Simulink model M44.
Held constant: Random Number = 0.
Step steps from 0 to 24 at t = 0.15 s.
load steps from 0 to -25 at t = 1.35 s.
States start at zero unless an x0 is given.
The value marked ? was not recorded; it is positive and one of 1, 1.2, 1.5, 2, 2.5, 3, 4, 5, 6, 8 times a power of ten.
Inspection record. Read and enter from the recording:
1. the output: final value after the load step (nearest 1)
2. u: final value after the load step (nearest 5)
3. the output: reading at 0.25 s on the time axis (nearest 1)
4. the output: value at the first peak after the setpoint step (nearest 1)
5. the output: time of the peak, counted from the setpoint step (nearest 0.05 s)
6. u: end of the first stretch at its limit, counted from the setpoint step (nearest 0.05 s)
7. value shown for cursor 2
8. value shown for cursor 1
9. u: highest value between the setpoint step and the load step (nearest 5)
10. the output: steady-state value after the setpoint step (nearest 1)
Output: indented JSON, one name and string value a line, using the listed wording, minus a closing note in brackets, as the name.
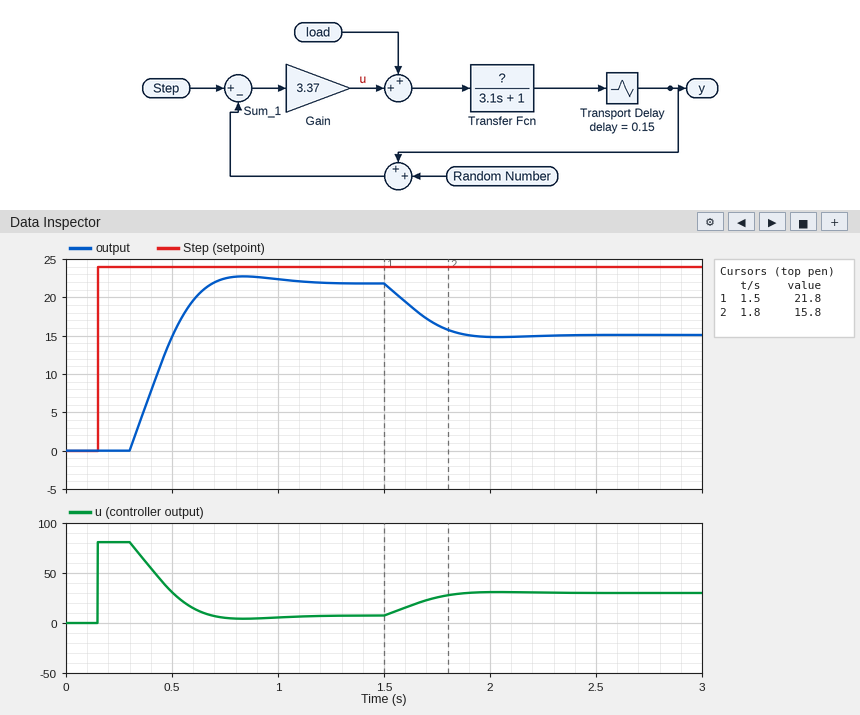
{
  "the output: final value after the load step": "15",
  "u: final value after the load step": "30",
  "the output: reading at 0.25 s on the time axis": "0",
  "the output: value at the first peak after the setpoint step": "23",
  "the output: time of the peak, counted from the setpoint step": "0.70 s",
  "u: end of the first stretch at its limit, counted from the setpoint step": "0.15 s",
  "value shown for cursor 2": "15.8",
  "value shown for cursor 1": "21.8",
  "u: highest value between the setpoint step and the load step": "80",
  "the output: steady-state value after the setpoint step": "22"
}
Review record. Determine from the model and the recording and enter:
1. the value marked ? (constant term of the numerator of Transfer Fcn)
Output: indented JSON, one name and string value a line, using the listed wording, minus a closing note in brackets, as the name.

{
  "the value marked ?": "3"
}
